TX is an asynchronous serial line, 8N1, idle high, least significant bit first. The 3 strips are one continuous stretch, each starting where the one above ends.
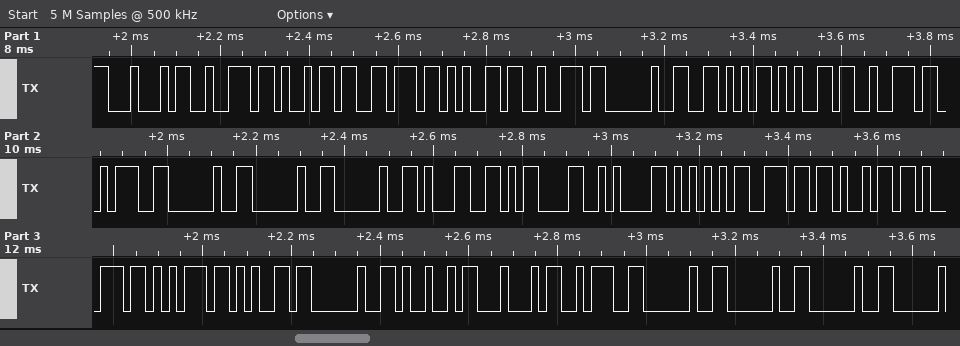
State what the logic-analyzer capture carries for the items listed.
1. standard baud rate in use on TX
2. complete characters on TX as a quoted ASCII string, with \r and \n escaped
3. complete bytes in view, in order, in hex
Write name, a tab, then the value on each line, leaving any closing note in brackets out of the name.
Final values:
standard baud rate in use on TX	57600 baud
complete characters on TX as a quoted ASCII string, with \r and \n escaped	"Driver Ver:   1\r\nUnique ID:   "
complete bytes in view, in order, in hex	44 72 69 76 65 72 20 56 65 72 3A 20 20 20 31 0D 0A 55 6E 69 71 75 65 20 49 44 3A 20 20 20
